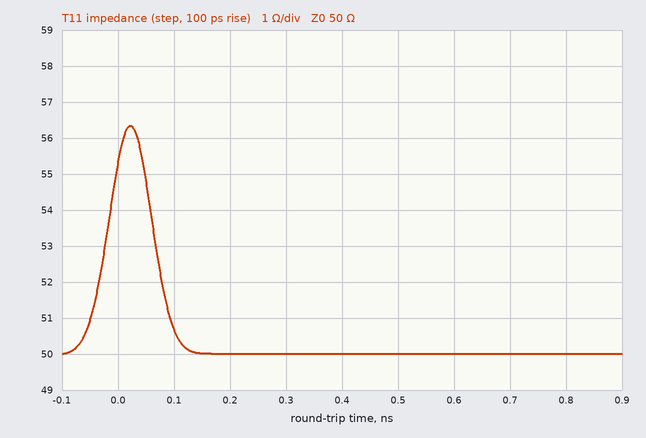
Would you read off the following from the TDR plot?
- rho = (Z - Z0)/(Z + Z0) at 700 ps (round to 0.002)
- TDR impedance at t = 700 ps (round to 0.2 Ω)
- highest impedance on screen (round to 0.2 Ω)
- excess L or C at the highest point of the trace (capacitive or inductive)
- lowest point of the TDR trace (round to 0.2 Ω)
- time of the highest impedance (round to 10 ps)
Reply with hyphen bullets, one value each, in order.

- 0.000
- 50.0 Ω
- 56.4 Ω
- inductive
- 50.0 Ω
- 20 ps
